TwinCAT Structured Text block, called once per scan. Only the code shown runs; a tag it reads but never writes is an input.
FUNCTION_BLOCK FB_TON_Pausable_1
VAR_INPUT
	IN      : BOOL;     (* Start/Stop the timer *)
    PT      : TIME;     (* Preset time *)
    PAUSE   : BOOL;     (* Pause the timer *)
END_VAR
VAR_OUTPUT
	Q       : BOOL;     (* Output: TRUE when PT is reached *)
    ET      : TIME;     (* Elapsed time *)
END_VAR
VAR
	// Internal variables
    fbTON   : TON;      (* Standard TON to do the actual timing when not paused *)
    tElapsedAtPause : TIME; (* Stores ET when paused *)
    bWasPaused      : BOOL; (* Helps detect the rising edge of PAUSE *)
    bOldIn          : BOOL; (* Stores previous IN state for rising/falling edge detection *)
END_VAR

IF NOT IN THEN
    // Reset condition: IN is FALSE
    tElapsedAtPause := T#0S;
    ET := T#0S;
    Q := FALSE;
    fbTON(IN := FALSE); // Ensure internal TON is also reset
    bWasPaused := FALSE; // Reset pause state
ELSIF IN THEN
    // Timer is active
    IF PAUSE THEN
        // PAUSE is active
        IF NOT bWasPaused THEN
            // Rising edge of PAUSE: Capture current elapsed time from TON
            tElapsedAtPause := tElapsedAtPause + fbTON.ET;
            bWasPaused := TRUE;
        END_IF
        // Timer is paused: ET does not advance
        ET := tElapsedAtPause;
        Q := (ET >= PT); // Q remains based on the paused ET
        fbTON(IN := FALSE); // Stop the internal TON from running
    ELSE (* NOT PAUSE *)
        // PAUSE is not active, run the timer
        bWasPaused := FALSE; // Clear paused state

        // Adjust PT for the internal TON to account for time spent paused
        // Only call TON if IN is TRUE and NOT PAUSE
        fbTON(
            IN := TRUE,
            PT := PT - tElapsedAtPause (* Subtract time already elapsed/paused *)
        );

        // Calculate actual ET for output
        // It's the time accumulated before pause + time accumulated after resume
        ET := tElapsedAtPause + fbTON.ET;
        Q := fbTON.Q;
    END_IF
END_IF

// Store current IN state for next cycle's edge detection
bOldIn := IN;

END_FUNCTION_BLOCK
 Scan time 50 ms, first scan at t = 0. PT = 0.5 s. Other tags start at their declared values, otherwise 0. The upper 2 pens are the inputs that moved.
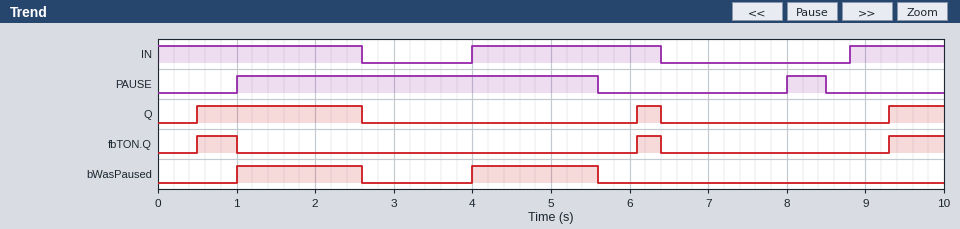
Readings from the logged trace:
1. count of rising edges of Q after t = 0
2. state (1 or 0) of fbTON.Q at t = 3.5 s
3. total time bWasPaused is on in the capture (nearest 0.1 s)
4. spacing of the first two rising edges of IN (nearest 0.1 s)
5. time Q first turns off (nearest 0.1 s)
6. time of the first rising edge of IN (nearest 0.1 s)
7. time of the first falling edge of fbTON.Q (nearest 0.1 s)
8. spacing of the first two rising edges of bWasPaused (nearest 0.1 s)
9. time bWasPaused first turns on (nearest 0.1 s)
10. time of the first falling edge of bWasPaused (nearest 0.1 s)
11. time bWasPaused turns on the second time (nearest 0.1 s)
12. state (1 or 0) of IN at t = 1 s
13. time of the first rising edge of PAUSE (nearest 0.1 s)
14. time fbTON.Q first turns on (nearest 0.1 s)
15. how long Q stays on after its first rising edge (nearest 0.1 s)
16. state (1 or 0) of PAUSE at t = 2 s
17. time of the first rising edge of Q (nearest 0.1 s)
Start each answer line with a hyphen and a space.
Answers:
- 3
- 0
- 3.2 s
- 4.8 s
- 2.6 s
- 4.0 s
- 1.0 s
- 3.0 s
- 1.0 s
- 2.6 s
- 4.0 s
- 1
- 1.0 s
- 0.5 s
- 2.1 s
- 1
- 0.5 s
